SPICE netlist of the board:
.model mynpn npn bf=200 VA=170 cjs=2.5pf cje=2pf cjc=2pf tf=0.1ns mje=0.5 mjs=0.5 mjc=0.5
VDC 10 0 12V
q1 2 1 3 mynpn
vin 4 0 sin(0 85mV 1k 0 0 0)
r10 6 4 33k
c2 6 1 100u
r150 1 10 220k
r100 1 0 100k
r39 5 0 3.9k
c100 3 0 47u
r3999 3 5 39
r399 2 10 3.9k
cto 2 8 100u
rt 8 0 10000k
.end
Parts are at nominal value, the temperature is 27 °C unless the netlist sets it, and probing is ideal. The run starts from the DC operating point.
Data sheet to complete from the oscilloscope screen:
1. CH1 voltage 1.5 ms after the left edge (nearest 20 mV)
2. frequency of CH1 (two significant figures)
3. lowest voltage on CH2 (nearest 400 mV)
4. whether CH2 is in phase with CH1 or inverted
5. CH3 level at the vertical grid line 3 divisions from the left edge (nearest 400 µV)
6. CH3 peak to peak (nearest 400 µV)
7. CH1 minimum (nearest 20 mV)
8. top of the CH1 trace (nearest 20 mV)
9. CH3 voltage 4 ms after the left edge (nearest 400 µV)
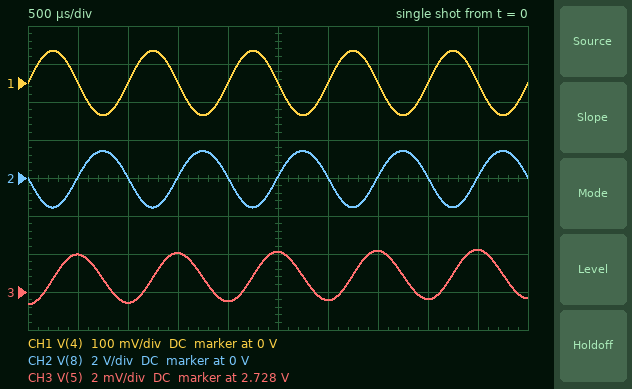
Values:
0 V
1.0 kHz
-1.6 V
inverted
2.7300 V
2.8 mV
-80 mV
80 mV
2.7276 V
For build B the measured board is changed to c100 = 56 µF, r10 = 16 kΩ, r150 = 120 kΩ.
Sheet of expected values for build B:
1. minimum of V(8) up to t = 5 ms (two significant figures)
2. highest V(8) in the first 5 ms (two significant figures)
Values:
-3.0 V
2.7 V
